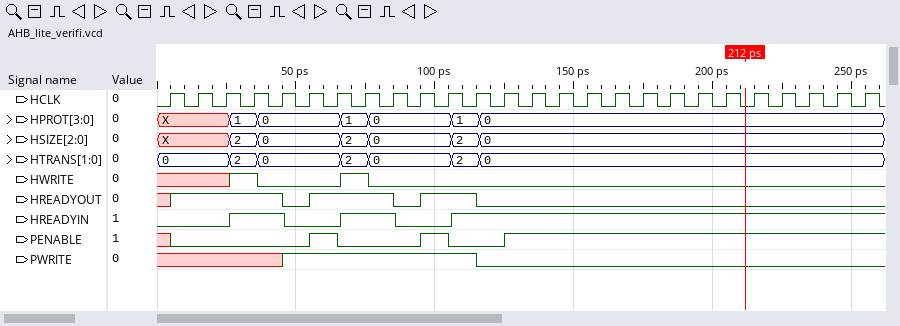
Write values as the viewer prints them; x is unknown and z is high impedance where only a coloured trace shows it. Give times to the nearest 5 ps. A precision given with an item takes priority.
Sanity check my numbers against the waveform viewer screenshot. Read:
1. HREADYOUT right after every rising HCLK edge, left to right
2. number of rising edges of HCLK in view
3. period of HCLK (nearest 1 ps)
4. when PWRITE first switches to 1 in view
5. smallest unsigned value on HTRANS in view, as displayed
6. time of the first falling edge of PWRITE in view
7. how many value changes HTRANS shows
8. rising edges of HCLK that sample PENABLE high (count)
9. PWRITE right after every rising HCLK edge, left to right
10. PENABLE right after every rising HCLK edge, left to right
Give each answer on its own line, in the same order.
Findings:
1 1 1 1 0 1 1 1 0 1 1 0 0 0 0 0 0 0 0 0 0 0 0 0 0 0
26
10 ps
45 ps
0
115 ps
6
15
x x x x 1 1 1 1 1 1 1 0 0 0 0 0 0 0 0 0 0 0 0 0 0 0
0 0 0 0 0 1 0 0 0 1 0 0 1 1 1 1 1 1 1 1 1 1 1 1 1 1
